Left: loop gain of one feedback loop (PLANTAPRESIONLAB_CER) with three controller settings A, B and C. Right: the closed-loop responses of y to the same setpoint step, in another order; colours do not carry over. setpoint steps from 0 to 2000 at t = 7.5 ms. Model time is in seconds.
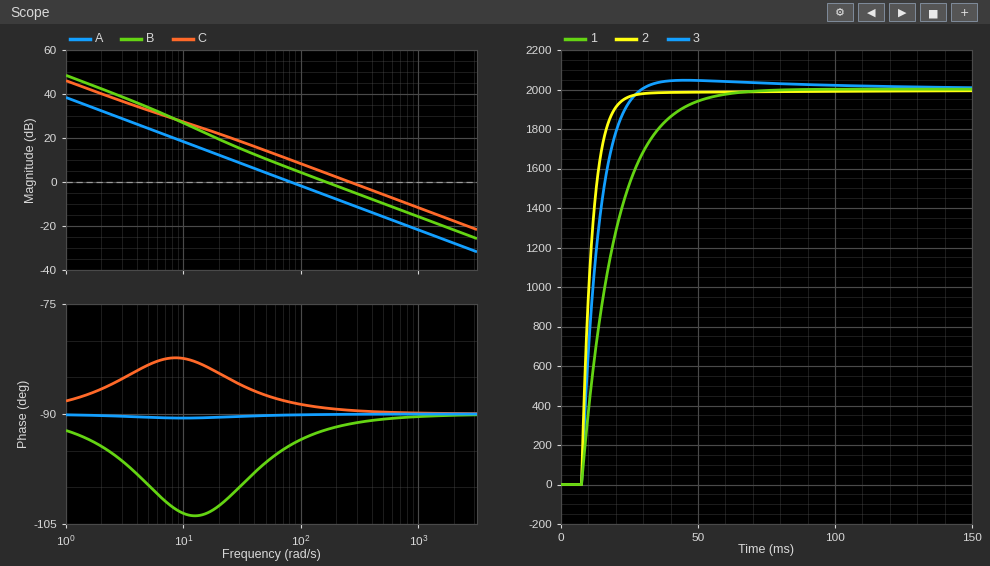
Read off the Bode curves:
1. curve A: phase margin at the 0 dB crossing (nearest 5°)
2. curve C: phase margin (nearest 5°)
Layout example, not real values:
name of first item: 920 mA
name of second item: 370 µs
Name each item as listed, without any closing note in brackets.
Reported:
curve A: phase margin at the 0 dB crossing: 90°
curve C: phase margin: 90°
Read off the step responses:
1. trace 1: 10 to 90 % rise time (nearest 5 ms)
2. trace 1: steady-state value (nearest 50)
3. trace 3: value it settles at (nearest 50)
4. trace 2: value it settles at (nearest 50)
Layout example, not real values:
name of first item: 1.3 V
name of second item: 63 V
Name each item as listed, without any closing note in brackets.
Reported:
trace 1: 10 to 90 % rise time: 25 ms
trace 1: steady-state value: 2000
trace 3: value it settles at: 2000
trace 2: value it settles at: 2000
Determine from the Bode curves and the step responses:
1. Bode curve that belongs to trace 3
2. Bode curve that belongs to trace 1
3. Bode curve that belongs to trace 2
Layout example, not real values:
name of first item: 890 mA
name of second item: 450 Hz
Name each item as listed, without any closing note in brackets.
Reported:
Bode curve that belongs to trace 3: B
Bode curve that belongs to trace 1: A
Bode curve that belongs to trace 2: C
